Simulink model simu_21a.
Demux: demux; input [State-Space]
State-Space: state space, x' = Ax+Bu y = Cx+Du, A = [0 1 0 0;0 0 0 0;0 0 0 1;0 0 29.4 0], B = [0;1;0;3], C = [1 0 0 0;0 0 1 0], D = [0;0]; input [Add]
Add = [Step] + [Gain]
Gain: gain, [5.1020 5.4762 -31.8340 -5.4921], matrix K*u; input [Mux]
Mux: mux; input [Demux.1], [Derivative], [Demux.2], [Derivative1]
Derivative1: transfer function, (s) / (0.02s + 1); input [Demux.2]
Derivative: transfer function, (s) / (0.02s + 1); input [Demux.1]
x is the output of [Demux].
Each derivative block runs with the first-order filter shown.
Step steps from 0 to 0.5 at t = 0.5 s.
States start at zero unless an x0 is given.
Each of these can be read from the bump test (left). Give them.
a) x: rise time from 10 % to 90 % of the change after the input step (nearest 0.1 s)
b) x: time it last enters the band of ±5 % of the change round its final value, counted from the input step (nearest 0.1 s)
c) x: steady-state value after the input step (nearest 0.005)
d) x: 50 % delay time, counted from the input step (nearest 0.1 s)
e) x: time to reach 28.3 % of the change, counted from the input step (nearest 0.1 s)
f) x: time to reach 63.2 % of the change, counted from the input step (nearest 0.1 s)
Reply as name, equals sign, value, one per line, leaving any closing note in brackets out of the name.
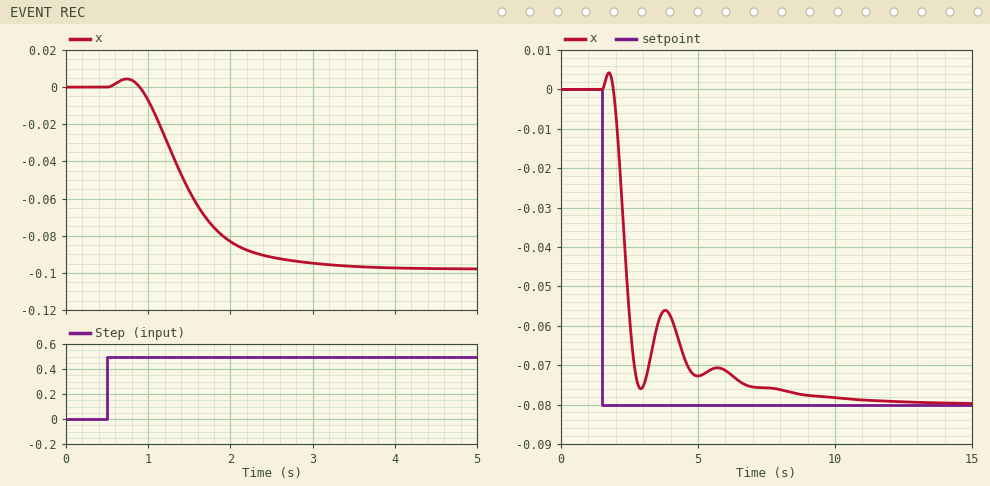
x: rise time from 10 % to 90 % of the change after the input step = 1.2 s
x: time it last enters the band of ±5 % of the change round its final value, counted from the input step = 2.2 s
x: steady-state value after the input step = -0.100
x: 50 % delay time, counted from the input step = 0.9 s
x: time to reach 28.3 % of the change, counted from the input step = 0.7 s
x: time to reach 63.2 % of the change, counted from the input step = 1.1 s
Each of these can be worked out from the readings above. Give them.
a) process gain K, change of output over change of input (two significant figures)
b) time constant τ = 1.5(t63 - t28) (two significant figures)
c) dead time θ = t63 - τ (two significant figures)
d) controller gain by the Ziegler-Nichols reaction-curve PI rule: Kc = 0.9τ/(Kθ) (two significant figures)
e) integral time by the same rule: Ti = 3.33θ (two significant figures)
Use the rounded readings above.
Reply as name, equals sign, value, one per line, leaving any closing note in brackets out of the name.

process gain K, change of output over change of input = -0.20
time constant τ = 1.5(t63 - t28) = 0.60 s
dead time θ = t63 - τ = 0.50 s
controller gain by the Ziegler-Nichols reaction-curve PI rule: Kc = 0.9τ/(Kθ) = -5.4
integral time by the same rule: Ti = 3.33θ = 1.7 s
